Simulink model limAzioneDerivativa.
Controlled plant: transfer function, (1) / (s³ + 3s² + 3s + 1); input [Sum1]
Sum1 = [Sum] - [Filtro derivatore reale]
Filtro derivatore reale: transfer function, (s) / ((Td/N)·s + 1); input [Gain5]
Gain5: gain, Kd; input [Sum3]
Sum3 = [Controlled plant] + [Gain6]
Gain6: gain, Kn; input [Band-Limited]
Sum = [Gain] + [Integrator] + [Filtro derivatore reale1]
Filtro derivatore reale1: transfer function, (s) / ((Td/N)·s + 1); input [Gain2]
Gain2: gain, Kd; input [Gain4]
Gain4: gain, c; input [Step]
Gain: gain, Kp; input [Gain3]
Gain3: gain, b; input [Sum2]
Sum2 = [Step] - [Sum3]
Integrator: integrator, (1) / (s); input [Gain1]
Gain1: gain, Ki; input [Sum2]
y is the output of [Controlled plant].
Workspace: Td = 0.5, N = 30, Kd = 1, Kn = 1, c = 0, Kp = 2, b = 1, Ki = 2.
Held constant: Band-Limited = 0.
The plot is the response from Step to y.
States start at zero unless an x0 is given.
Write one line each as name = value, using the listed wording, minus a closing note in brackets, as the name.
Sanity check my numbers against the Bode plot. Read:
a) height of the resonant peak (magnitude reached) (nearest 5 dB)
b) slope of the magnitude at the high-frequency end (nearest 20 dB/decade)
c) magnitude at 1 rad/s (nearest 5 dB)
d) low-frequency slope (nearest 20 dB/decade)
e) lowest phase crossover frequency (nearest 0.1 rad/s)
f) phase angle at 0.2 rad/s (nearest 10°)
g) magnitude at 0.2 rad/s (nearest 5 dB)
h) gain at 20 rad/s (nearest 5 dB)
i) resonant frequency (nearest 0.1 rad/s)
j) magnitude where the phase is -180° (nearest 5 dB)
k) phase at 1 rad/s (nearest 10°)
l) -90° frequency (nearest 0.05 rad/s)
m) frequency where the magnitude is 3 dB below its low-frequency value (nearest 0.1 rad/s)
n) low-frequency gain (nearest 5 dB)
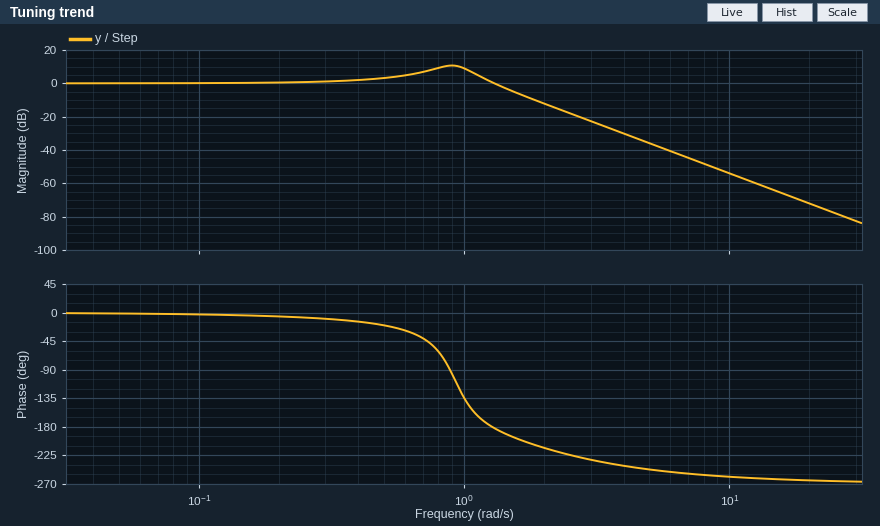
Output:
height of the resonant peak (magnitude reached) = 10 dB
slope of the magnitude at the high-frequency end = -60 dB/decade
magnitude at 1 rad/s = 10 dB
low-frequency slope = 0 dB/decade
lowest phase crossover frequency = 1.3 rad/s
phase angle at 0.2 rad/s = -10°
magnitude at 0.2 rad/s = 0 dB
gain at 20 rad/s = -70 dB
resonant frequency = 0.9 rad/s
magnitude where the phase is -180° = 0 dB
phase at 1 rad/s = -130°
-90° frequency = 0.90 rad/s
frequency where the magnitude is 3 dB below its low-frequency value = 1.4 rad/s
low-frequency gain = 0 dB
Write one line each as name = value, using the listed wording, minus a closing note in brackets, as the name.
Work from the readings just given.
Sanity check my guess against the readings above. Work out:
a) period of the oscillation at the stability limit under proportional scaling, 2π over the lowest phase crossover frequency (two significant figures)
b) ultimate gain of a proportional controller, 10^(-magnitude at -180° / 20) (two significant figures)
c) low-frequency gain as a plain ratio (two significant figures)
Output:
period of the oscillation at the stability limit under proportional scaling, 2π over the lowest phase crossover frequency = 4.8 s
ultimate gain of a proportional controller, 10^(-magnitude at -180° / 20) = 1.0
low-frequency gain as a plain ratio = 1.0
